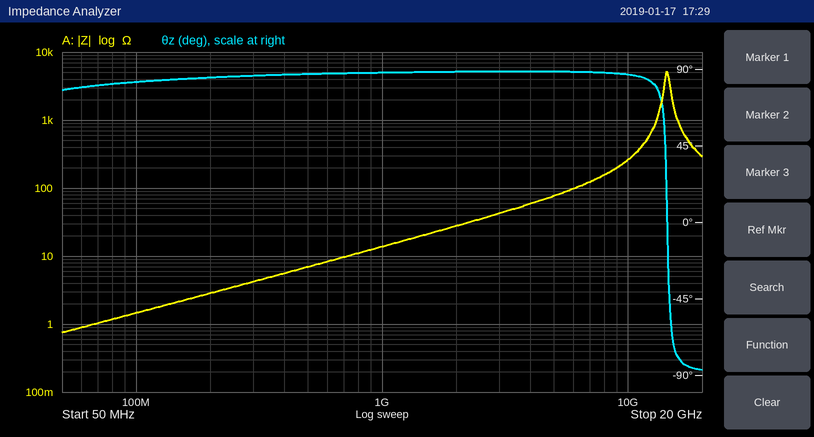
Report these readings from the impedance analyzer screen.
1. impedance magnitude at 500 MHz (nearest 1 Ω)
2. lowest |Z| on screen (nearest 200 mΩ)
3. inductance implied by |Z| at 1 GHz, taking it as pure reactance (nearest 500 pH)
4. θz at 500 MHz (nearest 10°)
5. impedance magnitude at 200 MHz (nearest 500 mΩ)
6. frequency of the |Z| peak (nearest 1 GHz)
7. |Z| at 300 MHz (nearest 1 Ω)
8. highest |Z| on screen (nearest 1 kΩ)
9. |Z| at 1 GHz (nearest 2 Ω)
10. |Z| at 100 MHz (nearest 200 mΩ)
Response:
7 Ω
800 mΩ
2.0 nH
90°
3.0 Ω
14 GHz
4 Ω
5 kΩ
14 Ω
1.4 Ω
